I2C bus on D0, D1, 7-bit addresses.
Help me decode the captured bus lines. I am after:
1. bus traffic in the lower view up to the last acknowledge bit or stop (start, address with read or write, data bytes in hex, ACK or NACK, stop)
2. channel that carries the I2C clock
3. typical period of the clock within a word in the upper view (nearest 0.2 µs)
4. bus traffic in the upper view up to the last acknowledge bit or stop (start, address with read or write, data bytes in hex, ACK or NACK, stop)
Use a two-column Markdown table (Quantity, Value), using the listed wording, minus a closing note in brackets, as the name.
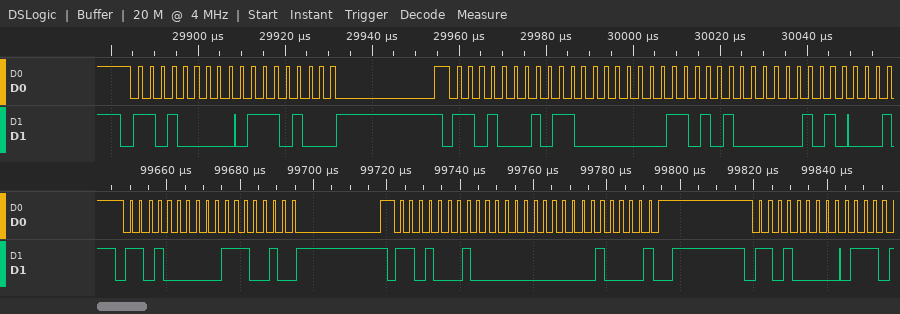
| Quantity | Value |
|---|---|
| bus traffic in the lower view up to the last acknowledge bit or stop | start, address 68 write ACK, 72 ACK, repeated start, address 68 read ACK, 00 ACK, 10 NACK, stop, start, address 68 write ACK |
| channel that carries the I2C clock | D0 |
| typical period of the clock within a word in the upper view | 2.6 µs |
| bus traffic in the upper view up to the last acknowledge bit or stop | start, address 68 write ACK, 74 ACK, repeated start, address 68 read ACK, C0 ACK, 6A ACK, 0A ACK |
